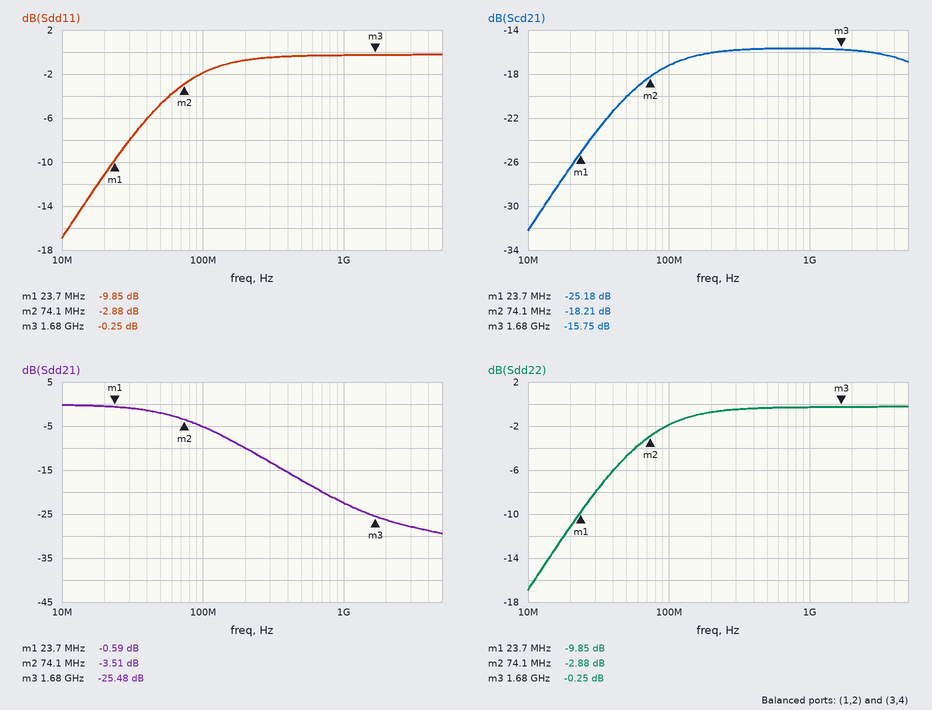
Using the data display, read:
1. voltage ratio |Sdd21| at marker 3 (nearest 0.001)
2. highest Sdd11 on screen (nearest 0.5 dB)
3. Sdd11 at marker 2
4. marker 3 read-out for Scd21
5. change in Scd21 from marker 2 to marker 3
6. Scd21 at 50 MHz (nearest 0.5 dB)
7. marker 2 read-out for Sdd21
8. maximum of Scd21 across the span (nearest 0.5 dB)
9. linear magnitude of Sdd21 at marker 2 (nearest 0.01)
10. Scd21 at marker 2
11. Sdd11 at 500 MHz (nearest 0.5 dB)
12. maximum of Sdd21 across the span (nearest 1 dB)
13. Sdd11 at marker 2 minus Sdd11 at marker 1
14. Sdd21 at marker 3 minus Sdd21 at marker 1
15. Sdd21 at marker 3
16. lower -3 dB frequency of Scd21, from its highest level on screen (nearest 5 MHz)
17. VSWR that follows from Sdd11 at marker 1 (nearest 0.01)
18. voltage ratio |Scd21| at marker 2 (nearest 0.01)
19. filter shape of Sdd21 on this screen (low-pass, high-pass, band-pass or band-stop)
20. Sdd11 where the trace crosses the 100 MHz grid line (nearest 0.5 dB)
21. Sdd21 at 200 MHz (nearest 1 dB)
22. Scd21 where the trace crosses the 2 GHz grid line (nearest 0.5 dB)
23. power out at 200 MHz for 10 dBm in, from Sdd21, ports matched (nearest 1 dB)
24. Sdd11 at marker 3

0.053
0.0 dB
-2.88 dB
-15.75 dB
2.46 dB
-20.0 dB
-3.51 dB
-15.5 dB
0.67
-18.21 dB
-0.5 dB
0 dB
6.97 dB
-24.89 dB
-25.48 dB
65 MHz
1.95
0.12
low-pass
-2.0 dB
-10 dB
-16.0 dB
0 dBm
-0.25 dB
